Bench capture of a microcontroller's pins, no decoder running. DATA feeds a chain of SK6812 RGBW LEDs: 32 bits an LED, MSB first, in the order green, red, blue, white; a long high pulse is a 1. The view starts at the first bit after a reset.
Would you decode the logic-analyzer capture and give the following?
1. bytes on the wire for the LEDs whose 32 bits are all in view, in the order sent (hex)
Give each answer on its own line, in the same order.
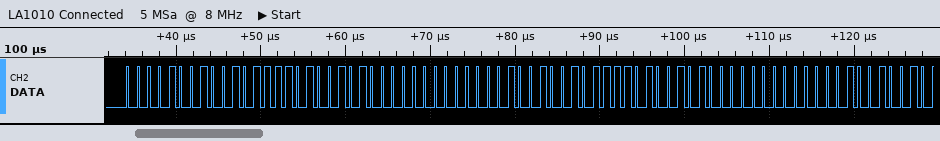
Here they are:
09 2F 4A 00 09 2F 4A 00
